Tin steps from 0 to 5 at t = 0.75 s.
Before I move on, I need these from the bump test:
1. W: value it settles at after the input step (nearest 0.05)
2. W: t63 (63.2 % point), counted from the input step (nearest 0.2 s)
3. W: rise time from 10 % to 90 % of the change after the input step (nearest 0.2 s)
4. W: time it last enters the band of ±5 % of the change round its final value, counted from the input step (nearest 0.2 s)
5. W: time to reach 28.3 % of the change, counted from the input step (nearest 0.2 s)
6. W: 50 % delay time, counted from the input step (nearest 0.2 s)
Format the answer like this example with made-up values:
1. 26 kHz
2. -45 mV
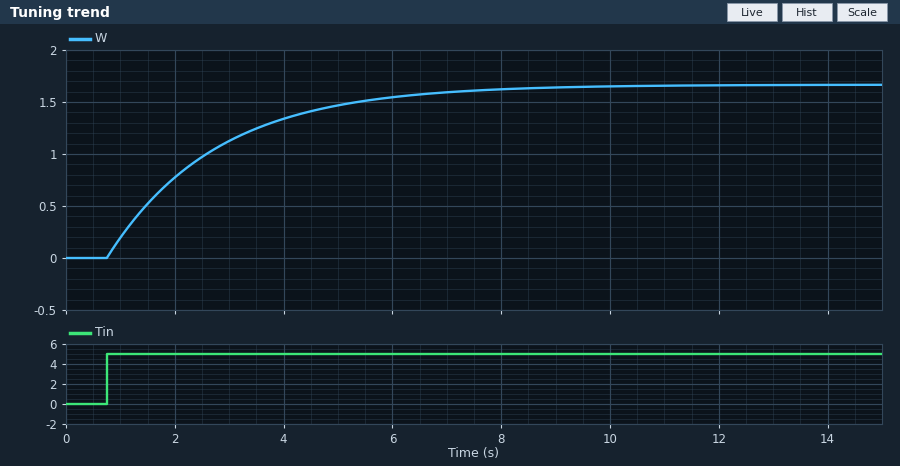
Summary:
1. 1.65
2. 2.0 s
3. 4.4 s
4. 6.0 s
5. 0.6 s
6. 1.4 s
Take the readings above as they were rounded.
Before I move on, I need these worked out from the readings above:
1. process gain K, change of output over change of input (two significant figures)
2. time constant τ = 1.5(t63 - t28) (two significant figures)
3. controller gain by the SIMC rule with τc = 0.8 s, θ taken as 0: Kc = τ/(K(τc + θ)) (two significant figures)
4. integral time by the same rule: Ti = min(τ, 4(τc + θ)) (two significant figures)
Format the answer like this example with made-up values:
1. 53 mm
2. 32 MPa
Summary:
1. 0.33
2. 2.1 s
3. 8.0
4. 2.1 s
